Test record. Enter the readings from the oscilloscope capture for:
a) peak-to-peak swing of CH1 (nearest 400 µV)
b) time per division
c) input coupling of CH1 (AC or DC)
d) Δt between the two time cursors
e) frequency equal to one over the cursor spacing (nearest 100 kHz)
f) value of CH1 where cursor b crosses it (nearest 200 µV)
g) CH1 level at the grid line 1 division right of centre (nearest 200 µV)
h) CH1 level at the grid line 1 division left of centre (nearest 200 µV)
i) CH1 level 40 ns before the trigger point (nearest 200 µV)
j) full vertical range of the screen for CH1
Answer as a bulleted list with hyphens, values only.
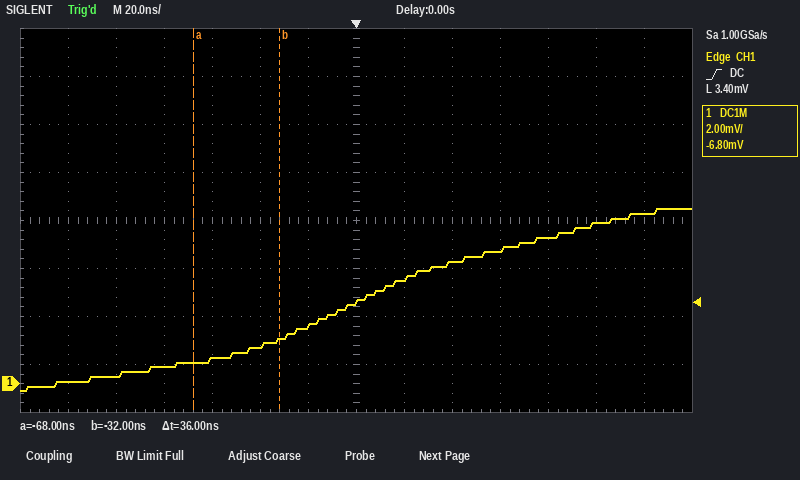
- 7.6 mV
- 20 ns
- DC
- 36 ns
- 27.8 MHz
- 1.8 mV
- 4.4 mV
- 2.4 mV
- 1.6 mV
- 16 mV
